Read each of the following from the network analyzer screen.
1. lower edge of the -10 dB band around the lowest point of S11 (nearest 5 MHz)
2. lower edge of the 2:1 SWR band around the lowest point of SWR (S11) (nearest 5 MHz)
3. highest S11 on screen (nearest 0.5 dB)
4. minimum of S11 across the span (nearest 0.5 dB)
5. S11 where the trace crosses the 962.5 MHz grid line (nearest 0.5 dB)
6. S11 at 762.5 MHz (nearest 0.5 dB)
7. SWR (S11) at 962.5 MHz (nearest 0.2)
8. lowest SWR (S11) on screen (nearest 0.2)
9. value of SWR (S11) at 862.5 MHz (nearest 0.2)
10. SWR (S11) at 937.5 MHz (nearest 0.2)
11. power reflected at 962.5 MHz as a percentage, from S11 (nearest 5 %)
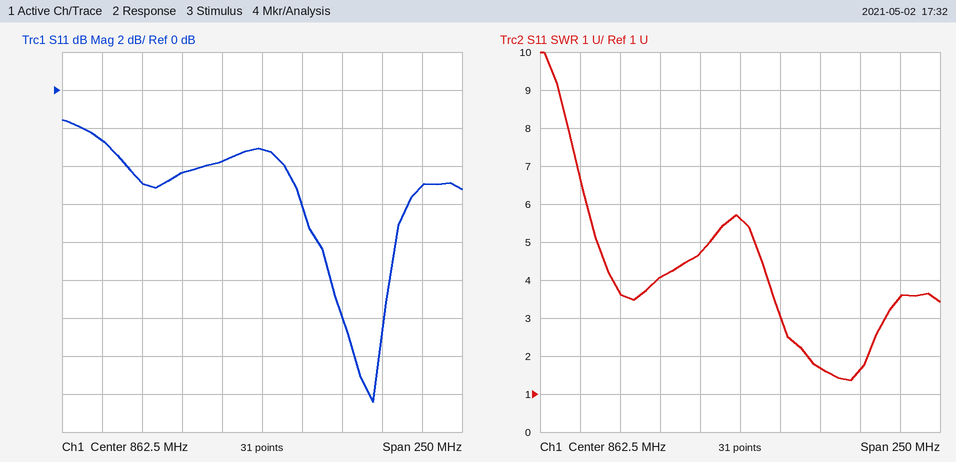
905 MHz
905 MHz
-1.5 dB
-16.5 dB
-5.0 dB
-2.5 dB
3.6
1.4
5.6
1.6
30 %
